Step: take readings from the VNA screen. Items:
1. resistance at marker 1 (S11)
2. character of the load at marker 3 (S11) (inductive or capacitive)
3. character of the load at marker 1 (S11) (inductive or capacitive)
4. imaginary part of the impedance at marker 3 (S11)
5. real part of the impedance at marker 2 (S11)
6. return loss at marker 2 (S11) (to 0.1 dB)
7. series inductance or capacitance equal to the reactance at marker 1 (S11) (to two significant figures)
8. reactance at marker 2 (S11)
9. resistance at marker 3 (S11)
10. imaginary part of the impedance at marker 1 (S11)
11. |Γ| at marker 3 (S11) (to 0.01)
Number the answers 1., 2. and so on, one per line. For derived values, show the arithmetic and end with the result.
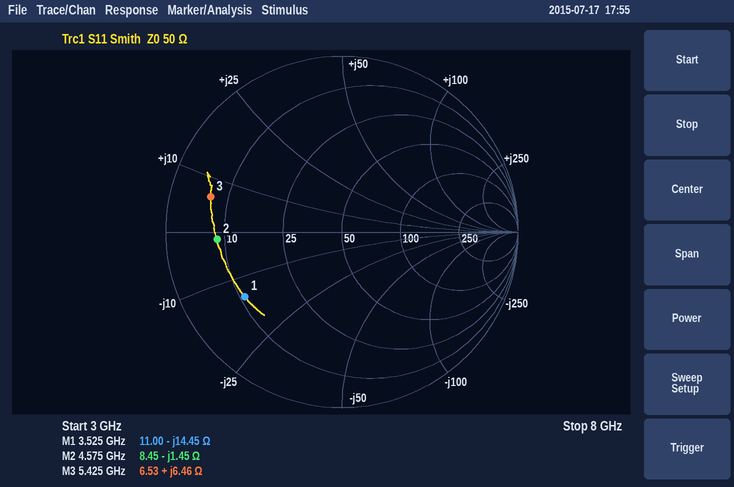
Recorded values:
1. 11.00 Ω
2. inductive
3. capacitive
4. +6.46 Ω
5. 8.45 Ω
6. 3.0 dB
7. C = 1/(2π × 3.525 GHz × 14.45 Ω) ≈ 3.1 pF
8. -1.45 Ω
9. 6.53 Ω
10. -14.45 Ω
11. 0.77
